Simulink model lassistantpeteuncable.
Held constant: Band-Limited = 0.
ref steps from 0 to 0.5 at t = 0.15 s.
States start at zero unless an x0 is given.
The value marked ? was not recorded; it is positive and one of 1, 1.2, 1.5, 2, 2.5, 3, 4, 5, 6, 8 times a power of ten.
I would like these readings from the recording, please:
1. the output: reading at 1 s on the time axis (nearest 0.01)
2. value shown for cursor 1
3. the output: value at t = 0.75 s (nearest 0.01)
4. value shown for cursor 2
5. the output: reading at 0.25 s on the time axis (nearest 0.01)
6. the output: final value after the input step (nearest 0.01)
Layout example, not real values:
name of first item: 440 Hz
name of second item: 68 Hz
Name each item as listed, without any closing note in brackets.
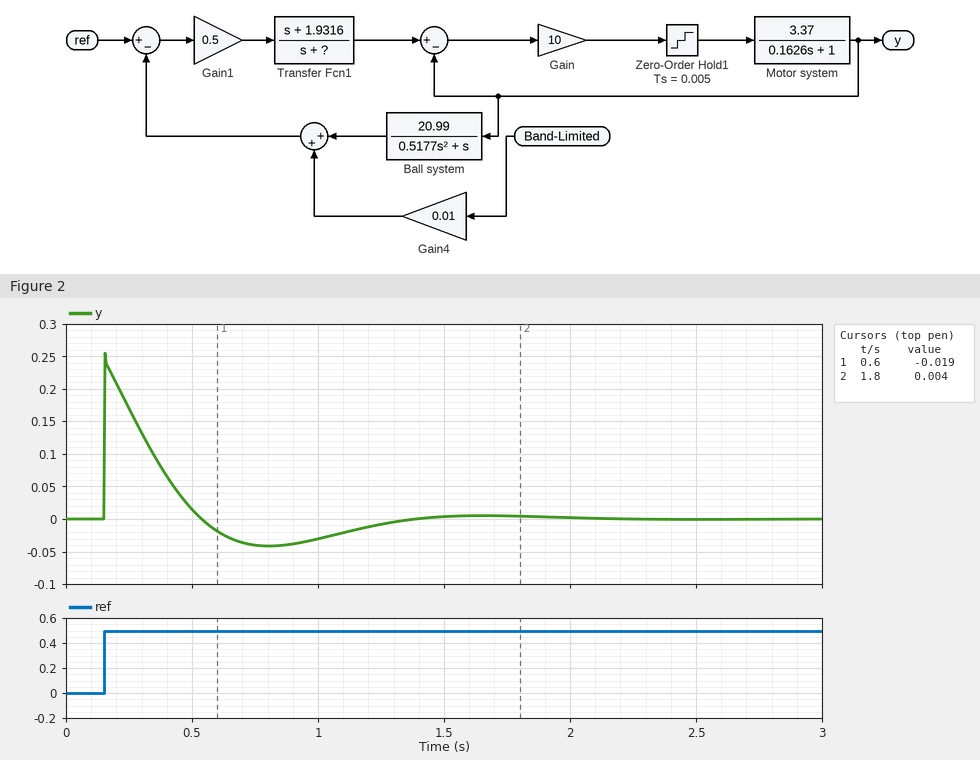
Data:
the output: reading at 1 s on the time axis: -0.03
value shown for cursor 1: -0.019
the output: value at t = 0.75 s: -0.04
value shown for cursor 2: 0.004
the output: reading at 0.25 s on the time axis: 0.17
the output: final value after the input step: 0.00
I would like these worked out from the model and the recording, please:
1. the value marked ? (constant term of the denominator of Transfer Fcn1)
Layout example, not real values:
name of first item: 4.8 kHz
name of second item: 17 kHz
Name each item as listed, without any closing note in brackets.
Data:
the value marked ?: 5
